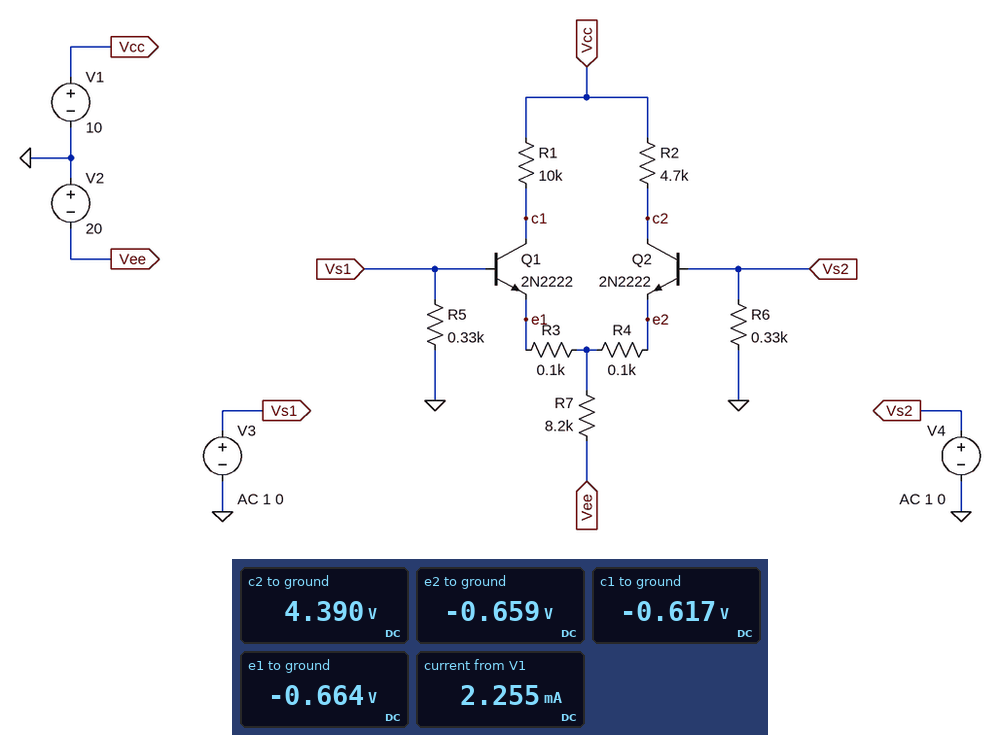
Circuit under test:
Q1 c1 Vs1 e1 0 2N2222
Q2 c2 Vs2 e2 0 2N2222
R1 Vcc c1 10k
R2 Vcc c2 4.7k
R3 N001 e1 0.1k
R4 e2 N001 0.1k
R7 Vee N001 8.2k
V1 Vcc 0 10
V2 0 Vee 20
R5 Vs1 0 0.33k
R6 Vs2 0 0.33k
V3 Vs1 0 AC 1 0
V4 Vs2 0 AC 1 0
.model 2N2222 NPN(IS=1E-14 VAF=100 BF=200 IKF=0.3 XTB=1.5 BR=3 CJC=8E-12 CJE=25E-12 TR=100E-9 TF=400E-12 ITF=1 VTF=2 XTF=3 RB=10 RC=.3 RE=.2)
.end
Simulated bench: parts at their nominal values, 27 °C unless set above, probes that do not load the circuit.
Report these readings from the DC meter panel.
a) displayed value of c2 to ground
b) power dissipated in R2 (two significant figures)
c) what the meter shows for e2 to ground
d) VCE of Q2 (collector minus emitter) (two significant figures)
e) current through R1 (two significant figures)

4.390 V
6.7 mW
-0.659 V
5.0 V
1.1 mA
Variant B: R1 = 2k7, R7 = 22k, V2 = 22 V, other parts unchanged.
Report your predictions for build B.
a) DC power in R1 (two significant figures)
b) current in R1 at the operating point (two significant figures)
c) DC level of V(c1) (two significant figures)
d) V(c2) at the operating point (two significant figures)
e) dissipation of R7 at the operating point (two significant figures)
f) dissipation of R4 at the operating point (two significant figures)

630 µW
480 µA
8.7 V
7.7 V
21 mW
23 µW
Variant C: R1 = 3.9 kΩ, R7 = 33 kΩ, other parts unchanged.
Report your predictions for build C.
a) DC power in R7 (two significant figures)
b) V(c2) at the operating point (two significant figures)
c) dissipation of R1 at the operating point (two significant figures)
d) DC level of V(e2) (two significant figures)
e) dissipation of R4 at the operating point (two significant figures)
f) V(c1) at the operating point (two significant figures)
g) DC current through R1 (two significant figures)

11 mW
8.6 V
330 µW
-620 mV
8.6 µW
8.9 V
290 µA
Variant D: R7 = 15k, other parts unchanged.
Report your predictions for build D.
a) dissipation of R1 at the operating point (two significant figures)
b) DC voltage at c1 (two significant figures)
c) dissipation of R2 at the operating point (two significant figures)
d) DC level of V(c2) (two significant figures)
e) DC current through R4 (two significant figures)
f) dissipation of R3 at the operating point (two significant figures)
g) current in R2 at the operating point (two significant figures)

4.1 mW
3.6 V
1.9 mW
7.0 V
650 µA
41 µW
640 µA
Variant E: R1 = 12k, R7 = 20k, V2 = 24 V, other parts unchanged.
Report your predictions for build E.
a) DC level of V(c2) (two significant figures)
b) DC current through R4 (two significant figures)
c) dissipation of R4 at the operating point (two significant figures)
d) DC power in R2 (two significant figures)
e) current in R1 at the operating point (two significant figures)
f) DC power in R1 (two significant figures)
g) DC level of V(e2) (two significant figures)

7.3 V
590 µA
34 µW
1.6 mW
580 µA
4.0 mW
-640 mV
